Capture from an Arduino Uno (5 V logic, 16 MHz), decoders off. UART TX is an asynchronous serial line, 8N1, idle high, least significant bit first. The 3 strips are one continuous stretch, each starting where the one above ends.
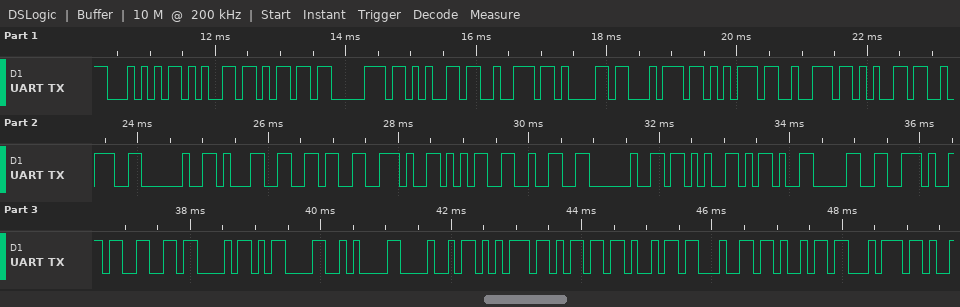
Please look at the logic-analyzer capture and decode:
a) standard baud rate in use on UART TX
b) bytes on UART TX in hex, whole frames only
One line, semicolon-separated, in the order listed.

9600 baud; 0x54 0x65 0x6D 0x70 0x65 0x72 0x61 0x74 0x75 0x72 0x65 0x3A 0x20 0x31 0x36 0x2E 0x35 0x32 0x20 0x2B 0x2D 0x30 0x2E 0x33 0x43 0x0D 0x0A 0x48 0x75 0x6D 0x69 0x64 0x69 0x74
